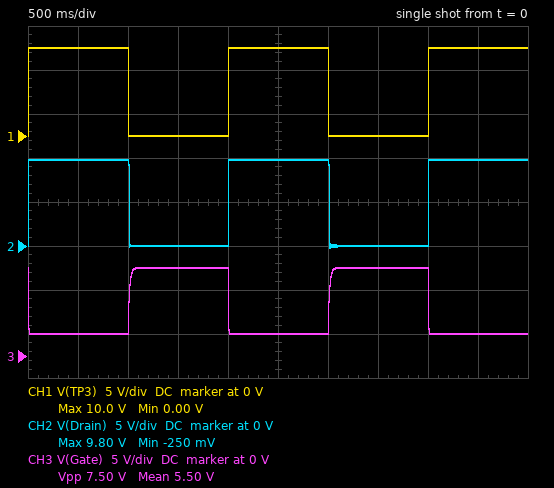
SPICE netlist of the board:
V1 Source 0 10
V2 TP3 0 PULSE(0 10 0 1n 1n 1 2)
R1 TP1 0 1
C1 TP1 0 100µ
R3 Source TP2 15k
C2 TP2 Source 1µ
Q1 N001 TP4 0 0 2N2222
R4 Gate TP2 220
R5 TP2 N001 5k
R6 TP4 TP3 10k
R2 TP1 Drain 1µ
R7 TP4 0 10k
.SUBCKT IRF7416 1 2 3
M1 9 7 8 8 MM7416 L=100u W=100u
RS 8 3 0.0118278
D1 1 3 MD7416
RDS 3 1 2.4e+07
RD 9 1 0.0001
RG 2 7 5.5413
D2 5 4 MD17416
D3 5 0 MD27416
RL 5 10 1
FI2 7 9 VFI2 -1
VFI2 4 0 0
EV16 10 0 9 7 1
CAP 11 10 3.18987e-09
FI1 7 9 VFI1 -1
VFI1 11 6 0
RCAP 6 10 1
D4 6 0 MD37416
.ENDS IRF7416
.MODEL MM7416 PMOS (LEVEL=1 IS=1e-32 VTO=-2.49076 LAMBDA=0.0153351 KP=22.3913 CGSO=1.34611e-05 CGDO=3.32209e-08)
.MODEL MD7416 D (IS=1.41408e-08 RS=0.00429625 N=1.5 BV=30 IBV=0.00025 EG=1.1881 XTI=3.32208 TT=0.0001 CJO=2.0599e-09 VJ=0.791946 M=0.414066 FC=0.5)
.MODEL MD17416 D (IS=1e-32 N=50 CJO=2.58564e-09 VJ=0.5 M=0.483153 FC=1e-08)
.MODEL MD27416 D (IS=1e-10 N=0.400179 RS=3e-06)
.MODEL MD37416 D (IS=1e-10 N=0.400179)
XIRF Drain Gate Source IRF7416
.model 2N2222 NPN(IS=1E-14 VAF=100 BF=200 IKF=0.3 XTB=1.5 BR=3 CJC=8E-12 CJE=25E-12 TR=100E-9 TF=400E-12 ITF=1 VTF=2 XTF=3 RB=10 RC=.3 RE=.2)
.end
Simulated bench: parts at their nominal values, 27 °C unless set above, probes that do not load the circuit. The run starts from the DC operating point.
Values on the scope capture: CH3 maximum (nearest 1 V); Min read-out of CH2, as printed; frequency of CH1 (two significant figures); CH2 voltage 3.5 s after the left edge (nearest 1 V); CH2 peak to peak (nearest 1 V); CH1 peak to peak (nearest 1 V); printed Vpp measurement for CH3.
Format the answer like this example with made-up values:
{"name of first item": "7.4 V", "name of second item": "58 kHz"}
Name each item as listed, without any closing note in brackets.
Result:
{"CH3 maximum": "10 V", "Min read-out of CH2, as printed": "-250 mV", "frequency of CH1": "500 mHz", "CH2 voltage 3.5 s after the left edge": "0 V", "CH2 peak to peak": "10 V", "CH1 peak to peak": "10 V", "printed Vpp measurement for CH3": "7.50 V"}
